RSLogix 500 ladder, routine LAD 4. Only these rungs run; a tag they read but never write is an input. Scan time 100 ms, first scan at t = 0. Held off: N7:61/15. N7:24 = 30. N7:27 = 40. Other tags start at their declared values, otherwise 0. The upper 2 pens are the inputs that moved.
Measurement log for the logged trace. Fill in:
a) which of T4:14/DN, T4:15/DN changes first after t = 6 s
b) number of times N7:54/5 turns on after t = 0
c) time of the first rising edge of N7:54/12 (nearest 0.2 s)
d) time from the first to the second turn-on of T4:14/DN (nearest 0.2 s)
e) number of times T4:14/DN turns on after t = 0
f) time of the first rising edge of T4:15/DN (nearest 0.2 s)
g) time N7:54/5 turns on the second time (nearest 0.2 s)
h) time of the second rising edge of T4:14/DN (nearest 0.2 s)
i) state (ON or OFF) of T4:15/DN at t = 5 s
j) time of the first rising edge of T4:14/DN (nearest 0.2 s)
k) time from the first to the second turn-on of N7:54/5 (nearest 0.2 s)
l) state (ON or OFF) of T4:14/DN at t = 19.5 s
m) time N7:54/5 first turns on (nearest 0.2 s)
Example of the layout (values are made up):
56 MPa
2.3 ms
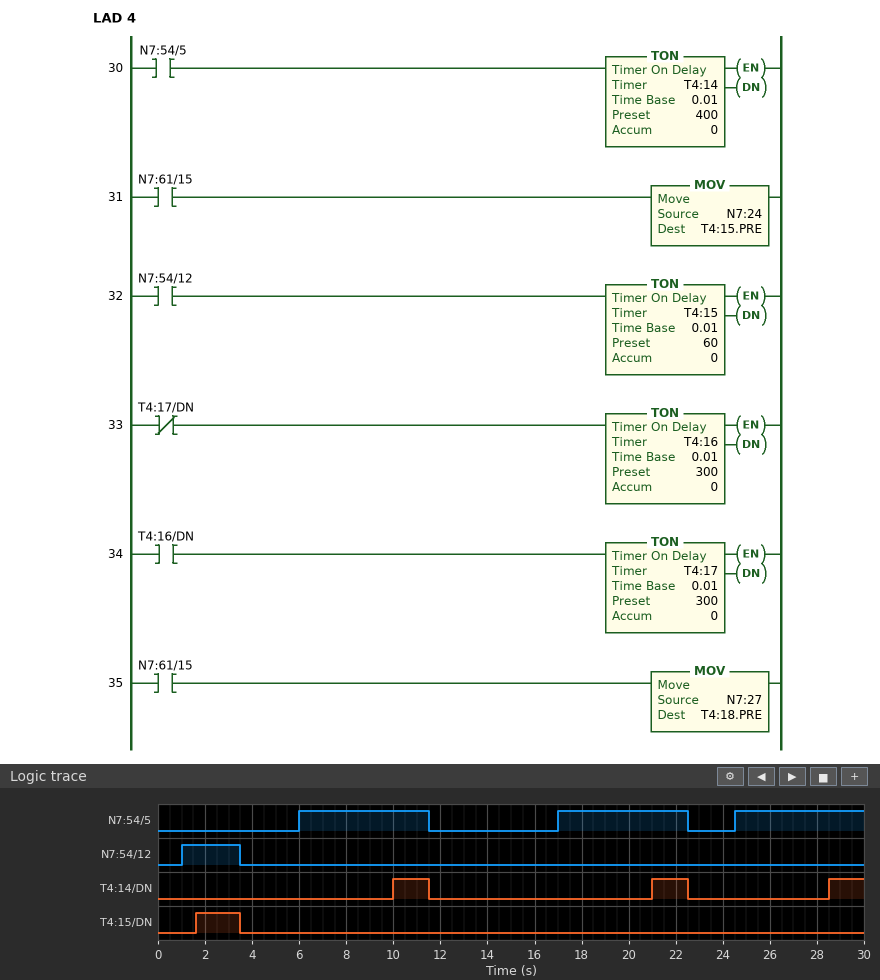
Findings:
T4:14/DN
3
1.0 s
11.0 s
3
1.6 s
17.0 s
21.0 s
OFF
10.0 s
11.0 s
OFF
6.0 s
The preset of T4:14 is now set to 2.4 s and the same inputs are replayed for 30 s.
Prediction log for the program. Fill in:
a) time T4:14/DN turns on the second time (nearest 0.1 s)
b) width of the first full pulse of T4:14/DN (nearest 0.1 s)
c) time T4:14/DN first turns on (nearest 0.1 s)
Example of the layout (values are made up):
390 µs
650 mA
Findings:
19.4 s
3.1 s
8.4 s
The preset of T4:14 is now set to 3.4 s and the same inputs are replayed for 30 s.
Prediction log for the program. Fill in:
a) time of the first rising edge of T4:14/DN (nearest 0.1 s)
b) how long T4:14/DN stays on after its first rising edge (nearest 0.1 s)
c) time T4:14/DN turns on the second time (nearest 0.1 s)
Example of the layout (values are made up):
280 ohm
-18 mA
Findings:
9.4 s
2.1 s
20.4 s
